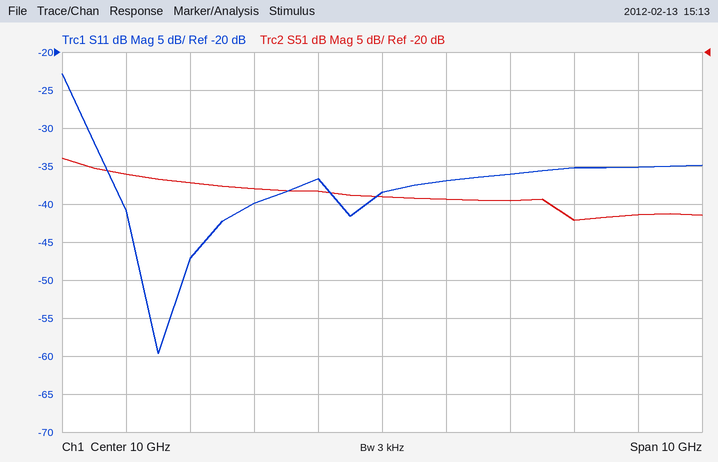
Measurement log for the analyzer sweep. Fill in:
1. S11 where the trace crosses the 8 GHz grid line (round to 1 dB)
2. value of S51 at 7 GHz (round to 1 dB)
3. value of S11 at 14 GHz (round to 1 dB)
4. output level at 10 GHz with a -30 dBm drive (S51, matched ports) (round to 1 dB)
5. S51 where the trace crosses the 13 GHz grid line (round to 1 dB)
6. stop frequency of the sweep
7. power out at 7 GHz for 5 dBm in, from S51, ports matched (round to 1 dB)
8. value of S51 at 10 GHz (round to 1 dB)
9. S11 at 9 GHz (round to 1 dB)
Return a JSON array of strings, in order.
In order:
["-40 dB", "-37 dB", "-35 dB", "-69 dBm", "-42 dB", "15 GHz", "-32 dBm", "-39 dB", "-37 dB"]
